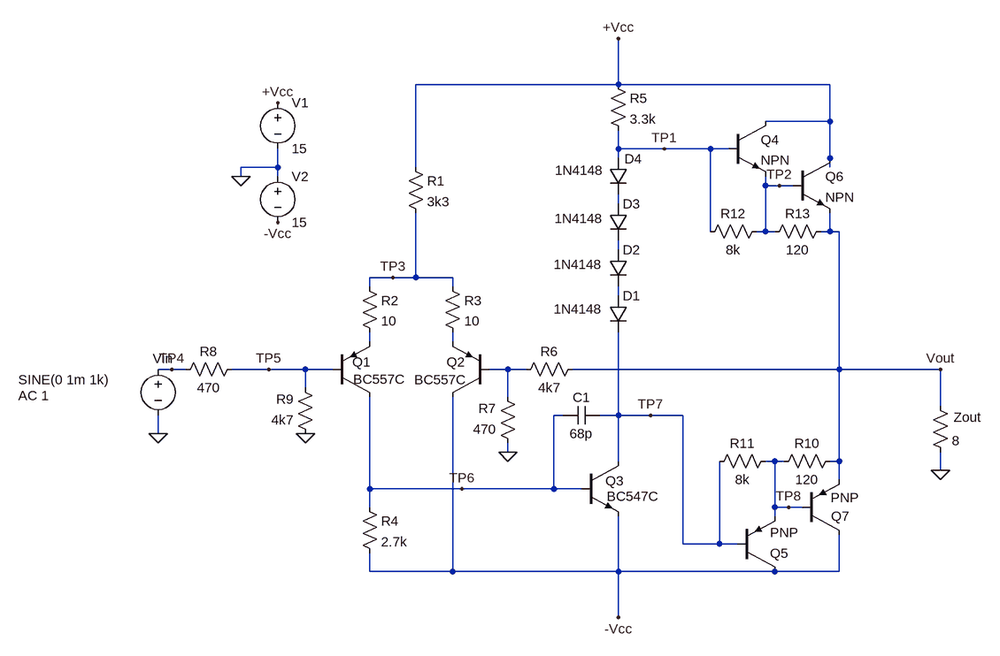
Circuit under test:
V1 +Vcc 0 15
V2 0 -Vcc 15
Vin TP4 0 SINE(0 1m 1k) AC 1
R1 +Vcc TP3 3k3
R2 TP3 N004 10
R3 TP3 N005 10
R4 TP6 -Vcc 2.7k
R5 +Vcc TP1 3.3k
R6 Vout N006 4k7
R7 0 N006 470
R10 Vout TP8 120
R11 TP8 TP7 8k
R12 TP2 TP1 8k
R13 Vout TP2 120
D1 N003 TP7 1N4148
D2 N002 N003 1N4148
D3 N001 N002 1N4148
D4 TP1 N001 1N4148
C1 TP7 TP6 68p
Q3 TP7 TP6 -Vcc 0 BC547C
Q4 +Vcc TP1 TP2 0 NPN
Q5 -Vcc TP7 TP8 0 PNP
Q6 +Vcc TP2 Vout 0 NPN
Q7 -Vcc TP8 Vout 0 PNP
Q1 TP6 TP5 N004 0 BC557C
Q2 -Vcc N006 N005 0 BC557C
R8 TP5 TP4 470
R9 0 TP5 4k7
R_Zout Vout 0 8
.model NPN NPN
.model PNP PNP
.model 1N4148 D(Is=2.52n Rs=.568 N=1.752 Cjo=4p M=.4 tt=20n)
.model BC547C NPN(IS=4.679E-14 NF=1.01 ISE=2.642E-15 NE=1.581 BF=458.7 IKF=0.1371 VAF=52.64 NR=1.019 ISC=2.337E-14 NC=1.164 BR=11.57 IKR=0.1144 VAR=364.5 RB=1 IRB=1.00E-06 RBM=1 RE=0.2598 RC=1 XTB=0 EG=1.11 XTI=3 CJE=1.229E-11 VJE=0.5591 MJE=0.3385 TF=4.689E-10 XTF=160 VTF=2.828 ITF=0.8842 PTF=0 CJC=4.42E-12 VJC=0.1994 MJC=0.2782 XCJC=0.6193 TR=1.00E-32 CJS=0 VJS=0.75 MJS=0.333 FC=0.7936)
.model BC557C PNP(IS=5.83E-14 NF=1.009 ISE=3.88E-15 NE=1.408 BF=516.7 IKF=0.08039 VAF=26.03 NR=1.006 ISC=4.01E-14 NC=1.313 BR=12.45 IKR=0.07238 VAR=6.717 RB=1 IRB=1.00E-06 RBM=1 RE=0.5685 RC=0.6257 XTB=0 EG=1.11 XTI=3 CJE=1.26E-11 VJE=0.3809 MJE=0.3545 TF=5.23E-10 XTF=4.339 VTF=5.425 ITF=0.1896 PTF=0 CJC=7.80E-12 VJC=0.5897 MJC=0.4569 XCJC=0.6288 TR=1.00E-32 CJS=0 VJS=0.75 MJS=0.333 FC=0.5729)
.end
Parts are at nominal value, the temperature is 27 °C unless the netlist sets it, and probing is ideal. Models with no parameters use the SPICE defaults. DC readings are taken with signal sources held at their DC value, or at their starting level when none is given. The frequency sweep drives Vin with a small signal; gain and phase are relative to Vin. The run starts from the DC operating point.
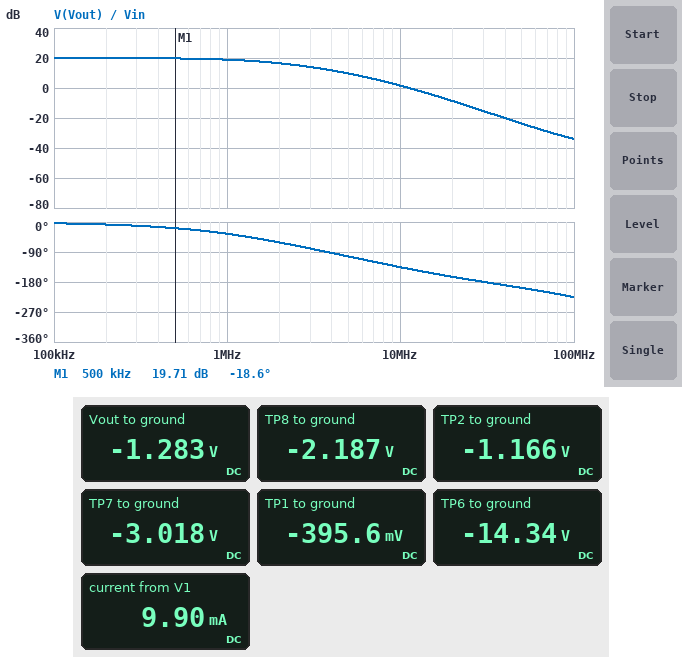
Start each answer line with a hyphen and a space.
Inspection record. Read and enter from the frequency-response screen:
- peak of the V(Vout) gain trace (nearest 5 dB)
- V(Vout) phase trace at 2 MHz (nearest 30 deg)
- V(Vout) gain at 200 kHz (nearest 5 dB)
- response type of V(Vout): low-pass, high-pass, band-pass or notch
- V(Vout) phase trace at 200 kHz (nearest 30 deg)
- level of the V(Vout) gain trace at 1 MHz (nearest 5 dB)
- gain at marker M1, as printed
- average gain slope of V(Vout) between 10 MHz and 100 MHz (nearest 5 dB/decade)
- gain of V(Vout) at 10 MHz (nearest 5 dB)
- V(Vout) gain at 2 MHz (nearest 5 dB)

- 20 dB
- -60 deg
- 20 dB
- low-pass
- 0 deg
- 20 dB
- 19.71 dB
- -35 dB/decade
- 0 dB
- 15 dB
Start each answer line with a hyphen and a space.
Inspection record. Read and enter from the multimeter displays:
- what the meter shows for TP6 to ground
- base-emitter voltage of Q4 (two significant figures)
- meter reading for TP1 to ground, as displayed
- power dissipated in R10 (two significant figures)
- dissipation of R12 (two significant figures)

- -14.34 V
- 770 mV
- -395.6 mV
- 6.8 mW
- 74 µW
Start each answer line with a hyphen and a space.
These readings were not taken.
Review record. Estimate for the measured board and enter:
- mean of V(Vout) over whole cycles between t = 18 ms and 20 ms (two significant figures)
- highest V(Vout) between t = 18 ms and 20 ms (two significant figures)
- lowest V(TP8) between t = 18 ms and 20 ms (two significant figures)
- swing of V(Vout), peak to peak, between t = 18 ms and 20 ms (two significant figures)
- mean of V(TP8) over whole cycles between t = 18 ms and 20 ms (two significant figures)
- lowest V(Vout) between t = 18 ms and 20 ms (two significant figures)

- -1.3 V
- -1.3 V
- -2.2 V
- 20 mV
- -2.2 V
- -1.3 V
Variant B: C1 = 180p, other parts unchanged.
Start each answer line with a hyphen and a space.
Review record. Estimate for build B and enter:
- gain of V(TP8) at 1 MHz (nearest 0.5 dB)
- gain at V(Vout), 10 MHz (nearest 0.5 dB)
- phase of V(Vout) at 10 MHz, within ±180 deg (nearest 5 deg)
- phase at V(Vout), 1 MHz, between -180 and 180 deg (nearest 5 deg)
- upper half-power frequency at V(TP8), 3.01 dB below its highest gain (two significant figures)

- 14.5 dB
- -7.0 dB
- -140 deg
- -65 deg
- 620 kHz
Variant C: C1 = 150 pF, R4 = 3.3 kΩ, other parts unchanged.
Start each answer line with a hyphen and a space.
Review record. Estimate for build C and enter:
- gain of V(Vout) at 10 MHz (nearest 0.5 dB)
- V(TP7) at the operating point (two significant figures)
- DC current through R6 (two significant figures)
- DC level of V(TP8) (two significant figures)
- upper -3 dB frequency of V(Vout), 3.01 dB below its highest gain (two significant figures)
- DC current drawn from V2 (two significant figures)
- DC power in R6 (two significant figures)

- -7.0 dB
- -3.1 V
- 260 µA
- -2.3 V
- 640 kHz
- 180 mA
- 320 µW
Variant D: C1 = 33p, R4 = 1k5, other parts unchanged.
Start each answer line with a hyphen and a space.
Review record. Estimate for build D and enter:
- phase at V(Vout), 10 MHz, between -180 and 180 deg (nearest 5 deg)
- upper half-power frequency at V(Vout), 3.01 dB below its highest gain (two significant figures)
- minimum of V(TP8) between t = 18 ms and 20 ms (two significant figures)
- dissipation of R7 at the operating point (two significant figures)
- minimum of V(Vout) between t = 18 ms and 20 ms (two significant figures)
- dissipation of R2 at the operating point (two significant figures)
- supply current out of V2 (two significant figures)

- -125 deg
- 6.7 MHz
- -2.0 V
- 19 µW
- -1.1 V
- 2.0 µW
- 140 mA
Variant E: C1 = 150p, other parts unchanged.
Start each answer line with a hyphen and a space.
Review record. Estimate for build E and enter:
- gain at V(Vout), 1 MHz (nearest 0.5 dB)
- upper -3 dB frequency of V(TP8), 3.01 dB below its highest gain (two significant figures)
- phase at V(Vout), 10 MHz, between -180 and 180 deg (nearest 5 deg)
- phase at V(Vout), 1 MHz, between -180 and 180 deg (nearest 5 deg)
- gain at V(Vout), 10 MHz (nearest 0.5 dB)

- 15.5 dB
- 750 kHz
- -140 deg
- -60 deg
- -5.5 dB
